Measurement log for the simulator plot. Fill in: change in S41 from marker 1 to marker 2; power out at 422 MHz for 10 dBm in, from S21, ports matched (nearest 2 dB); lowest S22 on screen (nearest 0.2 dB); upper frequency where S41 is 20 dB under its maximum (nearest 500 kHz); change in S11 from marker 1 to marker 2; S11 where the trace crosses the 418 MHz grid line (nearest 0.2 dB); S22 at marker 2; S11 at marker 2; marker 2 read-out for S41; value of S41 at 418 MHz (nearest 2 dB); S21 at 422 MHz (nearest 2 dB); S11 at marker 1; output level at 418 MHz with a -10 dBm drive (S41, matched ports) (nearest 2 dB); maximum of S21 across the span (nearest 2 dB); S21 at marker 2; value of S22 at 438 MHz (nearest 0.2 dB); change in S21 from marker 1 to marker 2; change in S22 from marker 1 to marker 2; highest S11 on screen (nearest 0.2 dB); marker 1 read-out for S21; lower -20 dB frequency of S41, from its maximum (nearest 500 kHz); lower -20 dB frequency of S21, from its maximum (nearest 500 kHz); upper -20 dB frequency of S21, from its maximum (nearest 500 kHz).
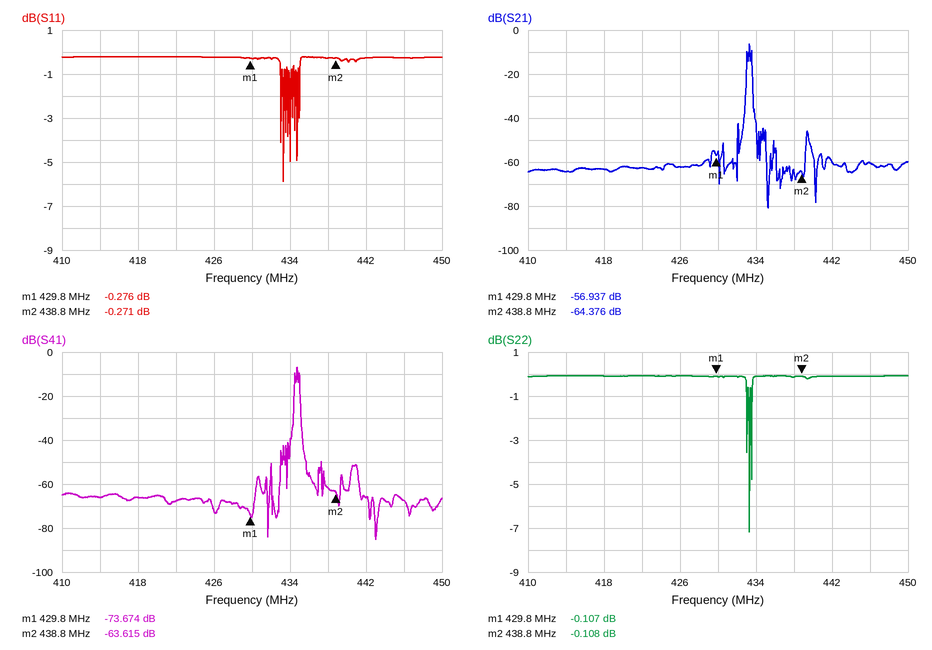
10.059 dB
-52 dBm
-7.2 dB
435.0 MHz
0.005 dB
-0.2 dB
-0.108 dB
-0.271 dB
-63.615 dB
-66 dB
-62 dB
-0.276 dB
-76 dBm
-6 dB
-64.376 dB
-0.2 dB
-7.439 dB
-0.001 dB
-0.2 dB
-56.937 dB
434.5 MHz
433.0 MHz
433.5 MHz
